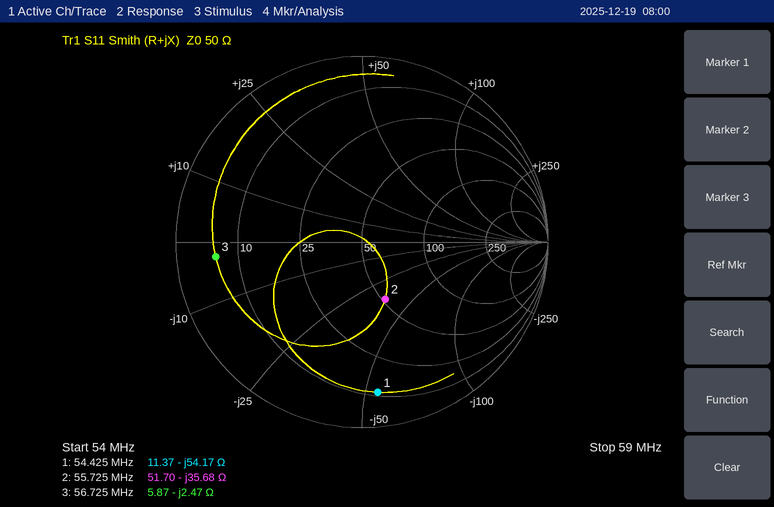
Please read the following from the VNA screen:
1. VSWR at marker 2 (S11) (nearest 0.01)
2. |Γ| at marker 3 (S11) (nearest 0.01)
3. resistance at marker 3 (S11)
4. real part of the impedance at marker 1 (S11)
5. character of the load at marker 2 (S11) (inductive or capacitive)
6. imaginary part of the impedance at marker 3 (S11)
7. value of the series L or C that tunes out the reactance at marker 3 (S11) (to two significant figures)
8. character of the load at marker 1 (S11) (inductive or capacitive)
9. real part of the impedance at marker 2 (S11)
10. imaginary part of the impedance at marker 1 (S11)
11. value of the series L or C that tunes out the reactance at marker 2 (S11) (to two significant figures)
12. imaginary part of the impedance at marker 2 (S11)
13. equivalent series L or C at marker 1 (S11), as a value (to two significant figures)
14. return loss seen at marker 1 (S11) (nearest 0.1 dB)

1.99
0.79
5.87 Ω
11.37 Ω
capacitive
-2.47 Ω
6.9 nH
capacitive
51.70 Ω
-54.17 Ω
100 nH
-35.68 Ω
54 pF
1.8 dB
